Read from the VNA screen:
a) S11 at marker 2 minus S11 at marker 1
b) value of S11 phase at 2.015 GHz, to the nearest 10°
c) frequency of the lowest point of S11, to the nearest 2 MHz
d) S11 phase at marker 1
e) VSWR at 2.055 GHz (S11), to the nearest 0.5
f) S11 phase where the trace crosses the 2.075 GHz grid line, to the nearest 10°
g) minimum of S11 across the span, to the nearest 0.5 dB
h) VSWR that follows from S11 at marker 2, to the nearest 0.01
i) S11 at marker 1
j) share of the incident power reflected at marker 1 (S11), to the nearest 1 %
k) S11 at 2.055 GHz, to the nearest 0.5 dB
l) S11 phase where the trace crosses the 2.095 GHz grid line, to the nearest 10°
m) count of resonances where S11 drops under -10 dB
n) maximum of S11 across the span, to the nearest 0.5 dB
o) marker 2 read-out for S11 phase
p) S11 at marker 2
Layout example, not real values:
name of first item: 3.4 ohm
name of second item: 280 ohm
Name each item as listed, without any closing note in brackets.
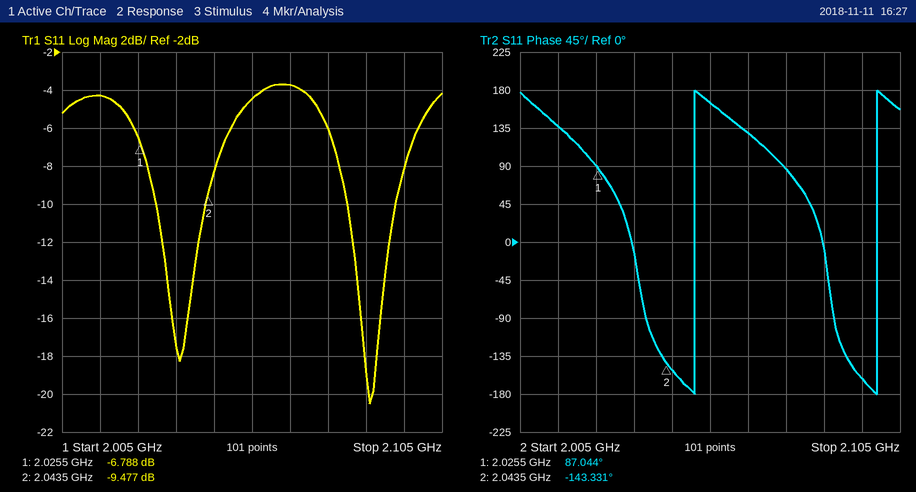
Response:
S11 at marker 2 minus S11 at marker 1: -2.689 dB
value of S11 phase at 2.015 GHz, to the nearest 10°: 140°
frequency of the lowest point of S11, to the nearest 2 MHz: 2.086 GHz
S11 phase at marker 1: 87.044°
VSWR at 2.055 GHz (S11), to the nearest 0.5: 4.0
S11 phase where the trace crosses the 2.075 GHz grid line, to the nearest 10°: 90°
minimum of S11 across the span, to the nearest 0.5 dB: -20.5 dB
VSWR that follows from S11 at marker 2, to the nearest 0.01: 2.01
S11 at marker 1: -6.788 dB
share of the incident power reflected at marker 1 (S11), to the nearest 1 %: 21 %
S11 at 2.055 GHz, to the nearest 0.5 dB: -4.5 dB
S11 phase where the trace crosses the 2.095 GHz grid line, to the nearest 10°: -160°
count of resonances where S11 drops under -10 dB: 2
maximum of S11 across the span, to the nearest 0.5 dB: -3.5 dB
marker 2 read-out for S11 phase: -143.331°
S11 at marker 2: -9.477 dB
